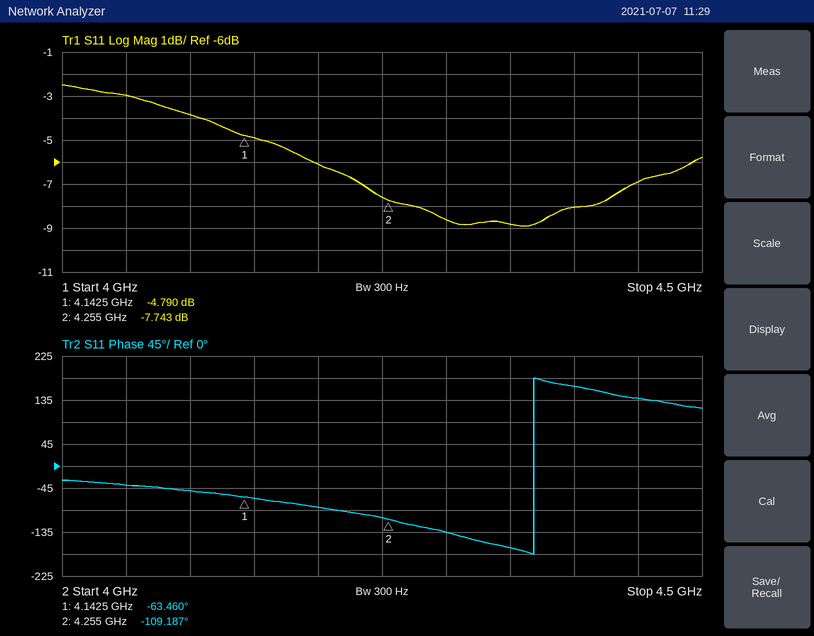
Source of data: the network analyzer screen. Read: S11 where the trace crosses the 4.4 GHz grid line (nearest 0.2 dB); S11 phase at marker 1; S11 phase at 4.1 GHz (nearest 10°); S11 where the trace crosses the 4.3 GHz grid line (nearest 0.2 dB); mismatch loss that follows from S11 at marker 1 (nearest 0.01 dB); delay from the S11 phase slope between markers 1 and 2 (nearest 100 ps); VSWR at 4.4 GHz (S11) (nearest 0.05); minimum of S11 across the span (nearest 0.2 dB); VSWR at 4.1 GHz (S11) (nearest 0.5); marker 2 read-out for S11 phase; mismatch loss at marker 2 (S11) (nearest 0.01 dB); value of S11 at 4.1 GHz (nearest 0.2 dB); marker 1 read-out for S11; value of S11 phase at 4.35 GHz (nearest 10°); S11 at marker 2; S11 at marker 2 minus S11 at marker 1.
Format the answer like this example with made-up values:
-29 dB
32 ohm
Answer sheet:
-8.0 dB
-63.460°
-50°
-8.6 dB
1.75 dB
1.1 ns
2.30
-9.0 dB
4.5
-109.187°
0.80 dB
-3.8 dB
-4.790 dB
-170°
-7.743 dB
-2.953 dB
